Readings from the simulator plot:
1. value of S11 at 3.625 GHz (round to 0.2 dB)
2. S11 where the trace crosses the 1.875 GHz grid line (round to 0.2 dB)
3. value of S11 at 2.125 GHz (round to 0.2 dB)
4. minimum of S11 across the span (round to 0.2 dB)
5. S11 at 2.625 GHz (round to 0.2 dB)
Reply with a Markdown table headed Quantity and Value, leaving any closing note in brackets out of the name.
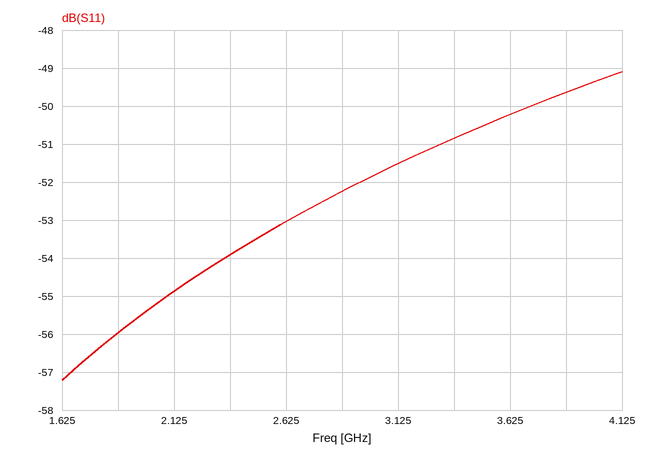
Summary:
| Quantity | Value |
|---|---|
| value of S11 at 3.625 GHz | -50.2 dB |
| S11 where the trace crosses the 1.875 GHz grid line | -56.0 dB |
| value of S11 at 2.125 GHz | -54.8 dB |
| minimum of S11 across the span | -57.2 dB |
| S11 at 2.625 GHz | -53.0 dB |
